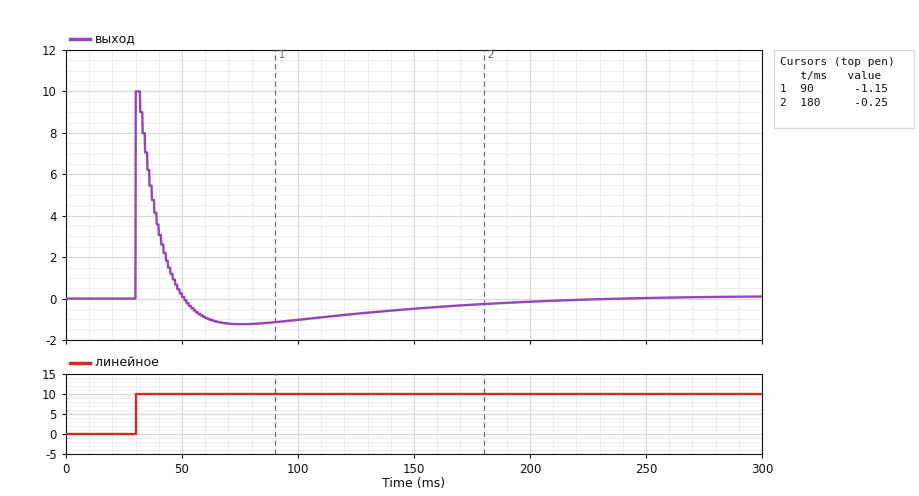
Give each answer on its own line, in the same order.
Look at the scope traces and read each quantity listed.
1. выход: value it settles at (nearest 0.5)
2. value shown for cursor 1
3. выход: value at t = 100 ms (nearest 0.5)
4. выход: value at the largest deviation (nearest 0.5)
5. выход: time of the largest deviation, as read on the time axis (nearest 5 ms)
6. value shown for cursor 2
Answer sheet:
0.0
-1.15
-1.0
10.0
30 ms
-0.25
